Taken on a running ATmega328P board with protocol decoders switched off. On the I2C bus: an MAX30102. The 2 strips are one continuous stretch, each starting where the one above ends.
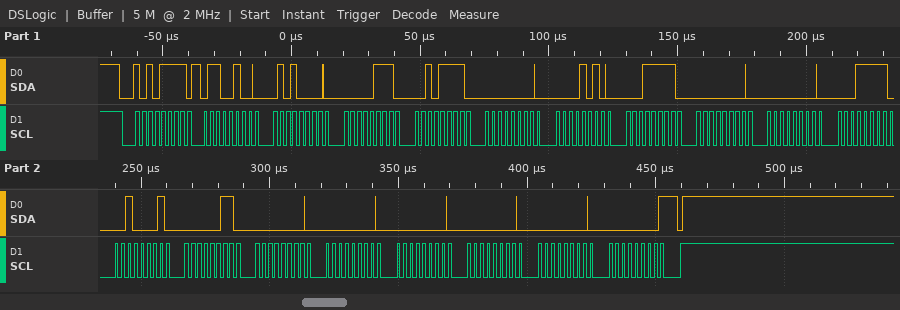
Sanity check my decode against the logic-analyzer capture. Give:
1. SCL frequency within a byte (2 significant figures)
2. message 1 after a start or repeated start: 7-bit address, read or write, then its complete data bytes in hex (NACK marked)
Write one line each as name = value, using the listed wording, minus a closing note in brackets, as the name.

SCL frequency within a byte = 400 kHz
message 1 after a start or repeated start: 7-bit address, read or write, then its complete data bytes in hex = 0x57 read: 64 50 07 2F 00 0A 1F 00 00 1F 21 03 00 00 00 00 00 00 NACK
